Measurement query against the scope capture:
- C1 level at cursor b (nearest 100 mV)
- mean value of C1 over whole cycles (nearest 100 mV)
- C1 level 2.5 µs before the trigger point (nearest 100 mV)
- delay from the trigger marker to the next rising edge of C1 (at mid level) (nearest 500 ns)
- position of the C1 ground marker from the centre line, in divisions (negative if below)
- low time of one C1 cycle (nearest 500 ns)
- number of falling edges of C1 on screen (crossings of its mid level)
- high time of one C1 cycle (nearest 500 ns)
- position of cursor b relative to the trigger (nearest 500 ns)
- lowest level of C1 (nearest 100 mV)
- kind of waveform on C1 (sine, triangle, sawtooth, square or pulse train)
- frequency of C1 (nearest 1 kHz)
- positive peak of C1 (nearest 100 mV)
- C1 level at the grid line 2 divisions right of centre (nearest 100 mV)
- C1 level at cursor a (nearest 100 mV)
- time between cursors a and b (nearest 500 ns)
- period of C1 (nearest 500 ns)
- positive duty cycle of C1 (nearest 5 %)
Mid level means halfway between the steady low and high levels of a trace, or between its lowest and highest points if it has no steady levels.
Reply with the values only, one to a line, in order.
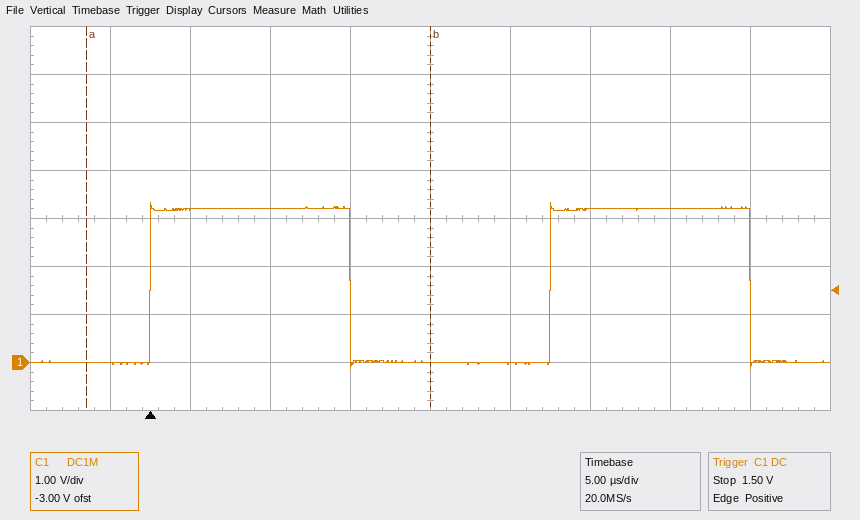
0.0 V
1.6 V
0.0 V
25.0 µs
-3.0 div
12.5 µs
2
12.5 µs
+17.5 µs
-100 mV
square
40 kHz
3.3 V
3.2 V
0.0 V
21.5 µs
25.0 µs
50 %
